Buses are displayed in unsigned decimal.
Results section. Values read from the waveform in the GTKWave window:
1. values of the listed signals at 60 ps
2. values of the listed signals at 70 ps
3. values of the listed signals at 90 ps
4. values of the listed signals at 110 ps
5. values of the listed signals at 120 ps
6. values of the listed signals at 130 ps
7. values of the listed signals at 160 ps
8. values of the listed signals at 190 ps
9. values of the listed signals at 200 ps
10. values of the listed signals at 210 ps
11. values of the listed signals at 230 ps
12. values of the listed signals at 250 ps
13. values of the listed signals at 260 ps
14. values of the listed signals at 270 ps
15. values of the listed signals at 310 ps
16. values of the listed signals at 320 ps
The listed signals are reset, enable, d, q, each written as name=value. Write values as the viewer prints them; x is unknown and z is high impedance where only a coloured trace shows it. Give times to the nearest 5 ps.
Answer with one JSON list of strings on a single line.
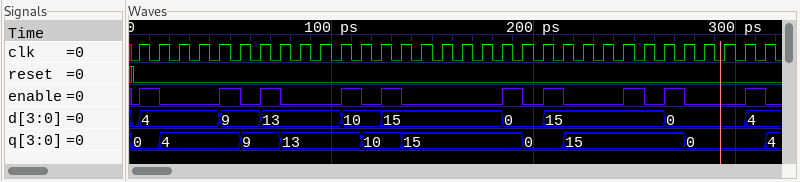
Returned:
["reset=0, enable=0, d=9, q=9", "reset=0, enable=1, d=13, q=9", "reset=0, enable=0, d=13, q=13", "reset=0, enable=1, d=10, q=13", "reset=0, enable=0, d=10, q=10", "reset=0, enable=1, d=15, q=10", "reset=0, enable=0, d=15, q=15", "reset=0, enable=1, d=0, q=15", "reset=0, enable=0, d=0, q=0", "reset=0, enable=1, d=15, q=0", "reset=0, enable=0, d=15, q=15", "reset=0, enable=1, d=15, q=15", "reset=0, enable=0, d=15, q=15", "reset=0, enable=1, d=0, q=15", "reset=0, enable=1, d=4, q=0", "reset=0, enable=0, d=4, q=4"]
